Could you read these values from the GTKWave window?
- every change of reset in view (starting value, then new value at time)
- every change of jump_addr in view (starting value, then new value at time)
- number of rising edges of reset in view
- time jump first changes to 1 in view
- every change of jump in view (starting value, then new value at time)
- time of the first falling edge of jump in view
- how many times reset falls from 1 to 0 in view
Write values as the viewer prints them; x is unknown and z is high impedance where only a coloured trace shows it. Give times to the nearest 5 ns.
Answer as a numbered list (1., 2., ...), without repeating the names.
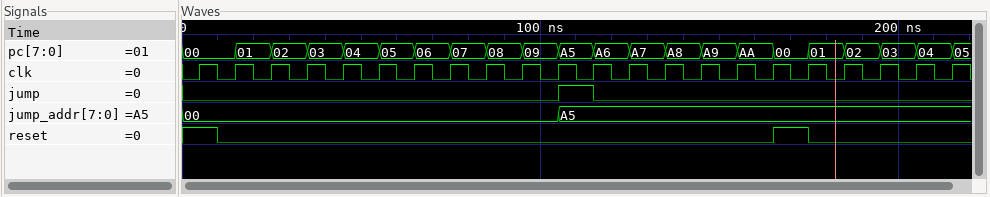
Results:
1. 1, 0 at 10 ns, 1 at 165 ns, 0 at 175 ns
2. 00, A5 at 105 ns
3. 1
4. 105 ns
5. 0, 1 at 105 ns, 0 at 115 ns
6. 115 ns
7. 2
